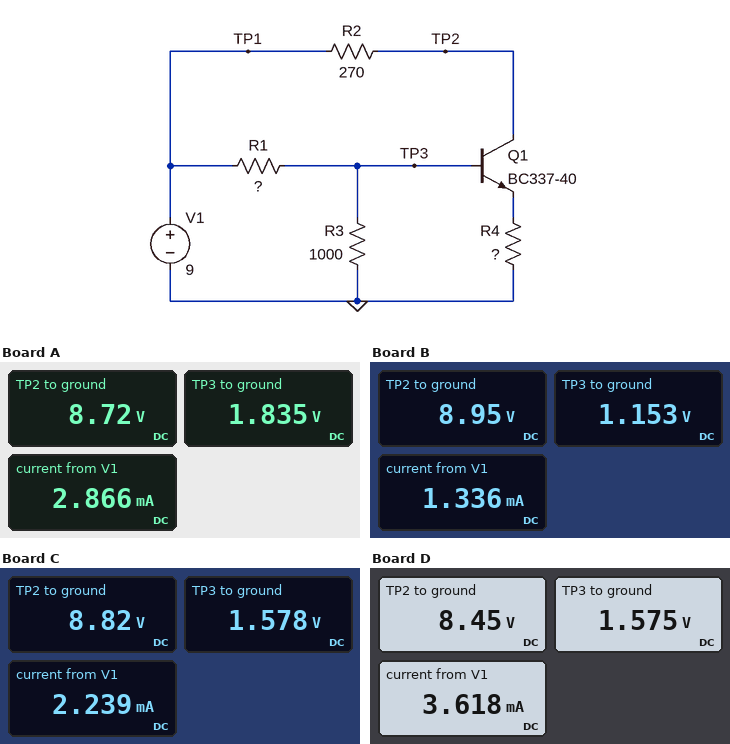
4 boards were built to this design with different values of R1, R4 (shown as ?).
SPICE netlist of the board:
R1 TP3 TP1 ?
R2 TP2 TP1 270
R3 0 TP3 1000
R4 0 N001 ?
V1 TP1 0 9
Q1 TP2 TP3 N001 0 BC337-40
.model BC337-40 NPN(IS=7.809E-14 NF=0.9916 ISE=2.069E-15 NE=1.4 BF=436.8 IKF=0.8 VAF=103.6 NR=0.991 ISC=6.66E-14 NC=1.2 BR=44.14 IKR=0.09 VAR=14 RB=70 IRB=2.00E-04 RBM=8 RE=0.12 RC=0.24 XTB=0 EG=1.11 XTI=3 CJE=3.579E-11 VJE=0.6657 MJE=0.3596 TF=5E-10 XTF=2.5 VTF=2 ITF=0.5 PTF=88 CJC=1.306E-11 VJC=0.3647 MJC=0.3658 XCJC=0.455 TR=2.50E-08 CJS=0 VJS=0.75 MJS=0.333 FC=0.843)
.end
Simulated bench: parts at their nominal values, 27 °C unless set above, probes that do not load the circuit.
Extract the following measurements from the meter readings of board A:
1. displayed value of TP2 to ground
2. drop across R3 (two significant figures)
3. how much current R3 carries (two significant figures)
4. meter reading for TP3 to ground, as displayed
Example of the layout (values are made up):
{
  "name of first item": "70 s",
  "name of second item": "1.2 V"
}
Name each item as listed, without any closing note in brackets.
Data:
{
  "displayed value of TP2 to ground": "8.72 V",
  "drop across R3": "1.8 V",
  "how much current R3 carries": "1.8 mA",
  "meter reading for TP3 to ground, as displayed": "1.835 V"
}
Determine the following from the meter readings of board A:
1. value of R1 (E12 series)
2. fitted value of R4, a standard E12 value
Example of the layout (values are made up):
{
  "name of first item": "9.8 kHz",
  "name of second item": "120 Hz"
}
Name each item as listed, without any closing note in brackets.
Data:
{
  "value of R1": "3.9 kΩ",
  "fitted value of R4, a standard E12 value": "1.2 kΩ"
}
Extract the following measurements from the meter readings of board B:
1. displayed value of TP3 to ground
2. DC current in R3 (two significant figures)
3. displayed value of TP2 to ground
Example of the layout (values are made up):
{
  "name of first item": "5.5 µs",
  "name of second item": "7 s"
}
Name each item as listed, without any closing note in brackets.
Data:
{
  "displayed value of TP3 to ground": "1.153 V",
  "DC current in R3": "1.2 mA",
  "displayed value of TP2 to ground": "8.95 V"
}
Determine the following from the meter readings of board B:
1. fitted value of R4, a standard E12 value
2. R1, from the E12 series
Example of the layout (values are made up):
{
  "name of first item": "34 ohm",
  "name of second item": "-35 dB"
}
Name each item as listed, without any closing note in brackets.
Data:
{
  "fitted value of R4, a standard E12 value": "3.3 kΩ",
  "R1, from the E12 series": "6.8 kΩ"
}
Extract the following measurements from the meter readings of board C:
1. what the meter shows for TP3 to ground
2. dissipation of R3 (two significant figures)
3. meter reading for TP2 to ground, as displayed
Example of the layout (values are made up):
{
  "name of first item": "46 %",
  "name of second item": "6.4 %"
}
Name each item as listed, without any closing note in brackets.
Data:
{
  "what the meter shows for TP3 to ground": "1.578 V",
  "dissipation of R3": "2.5 mW",
  "meter reading for TP2 to ground, as displayed": "8.82 V"
}
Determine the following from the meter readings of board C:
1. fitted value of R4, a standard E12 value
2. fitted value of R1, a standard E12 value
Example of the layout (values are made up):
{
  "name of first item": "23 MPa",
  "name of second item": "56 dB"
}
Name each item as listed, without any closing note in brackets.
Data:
{
  "fitted value of R4, a standard E12 value": "1.5 kΩ",
  "fitted value of R1, a standard E12 value": "4.7 kΩ"
}
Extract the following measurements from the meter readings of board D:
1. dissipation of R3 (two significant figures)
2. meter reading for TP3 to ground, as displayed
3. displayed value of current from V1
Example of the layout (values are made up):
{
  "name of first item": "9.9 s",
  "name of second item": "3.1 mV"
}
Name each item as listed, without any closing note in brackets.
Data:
{
  "dissipation of R3": "2.5 mW",
  "meter reading for TP3 to ground, as displayed": "1.575 V",
  "displayed value of current from V1": "3.618 mA"
}
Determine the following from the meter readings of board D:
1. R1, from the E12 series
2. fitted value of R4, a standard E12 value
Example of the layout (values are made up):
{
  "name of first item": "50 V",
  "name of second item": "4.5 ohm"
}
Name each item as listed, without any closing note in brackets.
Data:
{
  "R1, from the E12 series": "4.7 kΩ",
  "fitted value of R4, a standard E12 value": "470 Ω"
}
